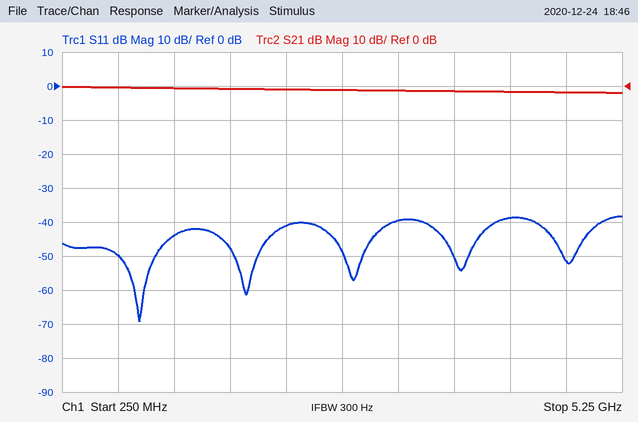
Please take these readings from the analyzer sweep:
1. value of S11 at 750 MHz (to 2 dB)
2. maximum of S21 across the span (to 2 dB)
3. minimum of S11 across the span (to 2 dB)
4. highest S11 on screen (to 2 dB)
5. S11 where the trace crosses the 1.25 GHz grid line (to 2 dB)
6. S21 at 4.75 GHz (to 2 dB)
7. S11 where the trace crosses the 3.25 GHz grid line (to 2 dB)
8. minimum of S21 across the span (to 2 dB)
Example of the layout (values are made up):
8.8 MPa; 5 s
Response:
-50 dB; 0 dB; -70 dB; -38 dB; -44 dB; -2 dB; -40 dB; -2 dB
